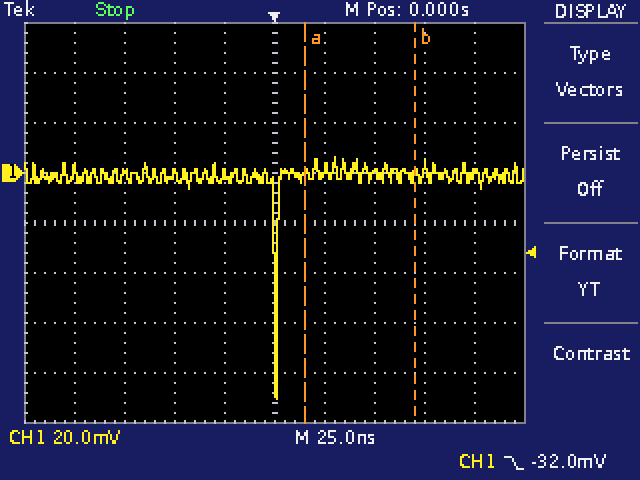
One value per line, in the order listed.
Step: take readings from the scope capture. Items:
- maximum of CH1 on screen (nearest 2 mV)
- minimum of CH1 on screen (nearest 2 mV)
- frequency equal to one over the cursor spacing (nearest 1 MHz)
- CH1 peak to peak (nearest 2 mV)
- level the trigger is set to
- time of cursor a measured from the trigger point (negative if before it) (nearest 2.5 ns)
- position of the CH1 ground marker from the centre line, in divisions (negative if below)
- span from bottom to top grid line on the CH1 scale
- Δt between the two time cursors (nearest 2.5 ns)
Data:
6 mV
-90 mV
18 MHz
96 mV
-32.0 mV
+15.0 ns
+1.0 div
160 mV
55.0 ns
